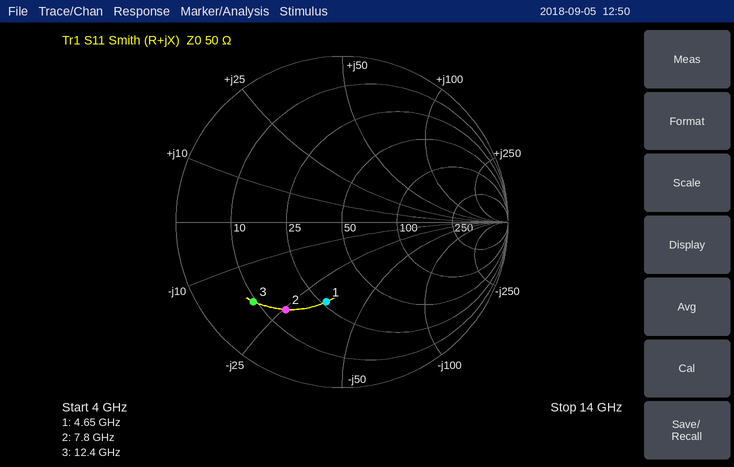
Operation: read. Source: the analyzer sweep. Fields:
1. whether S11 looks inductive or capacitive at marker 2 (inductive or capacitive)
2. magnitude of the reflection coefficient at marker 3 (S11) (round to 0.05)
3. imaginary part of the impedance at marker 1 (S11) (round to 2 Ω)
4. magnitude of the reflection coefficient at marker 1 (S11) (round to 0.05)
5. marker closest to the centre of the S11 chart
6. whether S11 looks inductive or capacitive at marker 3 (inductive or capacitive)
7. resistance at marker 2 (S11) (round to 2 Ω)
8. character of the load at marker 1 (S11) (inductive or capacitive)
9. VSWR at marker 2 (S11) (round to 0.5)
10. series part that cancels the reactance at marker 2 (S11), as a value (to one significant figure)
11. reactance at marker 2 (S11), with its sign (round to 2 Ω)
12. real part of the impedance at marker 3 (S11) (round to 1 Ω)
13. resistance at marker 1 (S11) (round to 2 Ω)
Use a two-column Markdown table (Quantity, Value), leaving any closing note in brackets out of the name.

| Quantity | Value |
|---|---|
| whether S11 looks inductive or capacitive at marker 2 | capacitive |
| magnitude of the reflection coefficient at marker 3 (S11) | 0.70 |
| imaginary part of the impedance at marker 1 (S11) | -34 Ω |
| magnitude of the reflection coefficient at marker 1 (S11) | 0.50 |
| marker closest to the centre of the S11 chart | marker 1 |
| whether S11 looks inductive or capacitive at marker 3 | capacitive |
| resistance at marker 2 (S11) | 14 Ω |
| character of the load at marker 1 (S11) | capacitive |
| VSWR at marker 2 (S11) | 4.5 |
| series part that cancels the reactance at marker 2 (S11), as a value | 500 pH |
| reactance at marker 2 (S11), with its sign | -26 Ω |
| real part of the impedance at marker 3 (S11) | 9 Ω |
| resistance at marker 1 (S11) | 26 Ω |
